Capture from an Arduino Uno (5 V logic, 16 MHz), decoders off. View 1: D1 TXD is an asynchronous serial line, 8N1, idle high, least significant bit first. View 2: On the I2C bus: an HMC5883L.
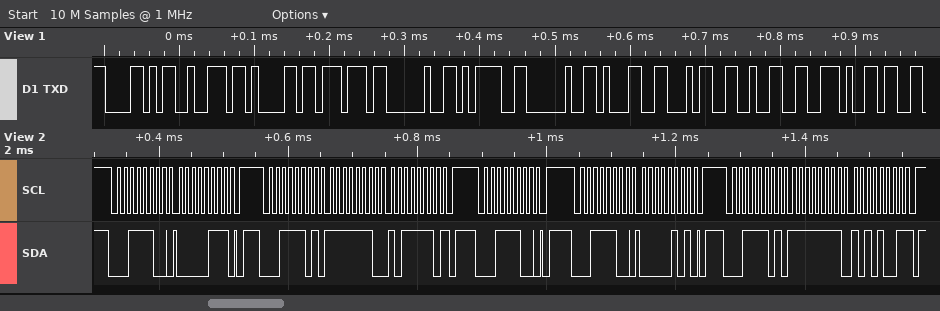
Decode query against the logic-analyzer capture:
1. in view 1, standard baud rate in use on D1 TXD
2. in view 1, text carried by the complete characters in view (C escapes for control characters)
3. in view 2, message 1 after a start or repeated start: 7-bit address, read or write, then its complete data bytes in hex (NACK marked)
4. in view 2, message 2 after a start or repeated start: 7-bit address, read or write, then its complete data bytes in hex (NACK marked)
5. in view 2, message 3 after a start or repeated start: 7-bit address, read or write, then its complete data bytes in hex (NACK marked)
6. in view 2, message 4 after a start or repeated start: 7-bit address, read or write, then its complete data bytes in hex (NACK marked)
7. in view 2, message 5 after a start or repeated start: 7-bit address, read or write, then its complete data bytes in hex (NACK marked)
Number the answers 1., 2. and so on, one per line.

1. 115200 baud
2. "Xraw = 142."
3. 0x1E write: 07
4. 0x1E read: FE BE NACK
5. 0x1E write
6. 0x1E write: 05
7. 0x1E read: FF A9 NACK
